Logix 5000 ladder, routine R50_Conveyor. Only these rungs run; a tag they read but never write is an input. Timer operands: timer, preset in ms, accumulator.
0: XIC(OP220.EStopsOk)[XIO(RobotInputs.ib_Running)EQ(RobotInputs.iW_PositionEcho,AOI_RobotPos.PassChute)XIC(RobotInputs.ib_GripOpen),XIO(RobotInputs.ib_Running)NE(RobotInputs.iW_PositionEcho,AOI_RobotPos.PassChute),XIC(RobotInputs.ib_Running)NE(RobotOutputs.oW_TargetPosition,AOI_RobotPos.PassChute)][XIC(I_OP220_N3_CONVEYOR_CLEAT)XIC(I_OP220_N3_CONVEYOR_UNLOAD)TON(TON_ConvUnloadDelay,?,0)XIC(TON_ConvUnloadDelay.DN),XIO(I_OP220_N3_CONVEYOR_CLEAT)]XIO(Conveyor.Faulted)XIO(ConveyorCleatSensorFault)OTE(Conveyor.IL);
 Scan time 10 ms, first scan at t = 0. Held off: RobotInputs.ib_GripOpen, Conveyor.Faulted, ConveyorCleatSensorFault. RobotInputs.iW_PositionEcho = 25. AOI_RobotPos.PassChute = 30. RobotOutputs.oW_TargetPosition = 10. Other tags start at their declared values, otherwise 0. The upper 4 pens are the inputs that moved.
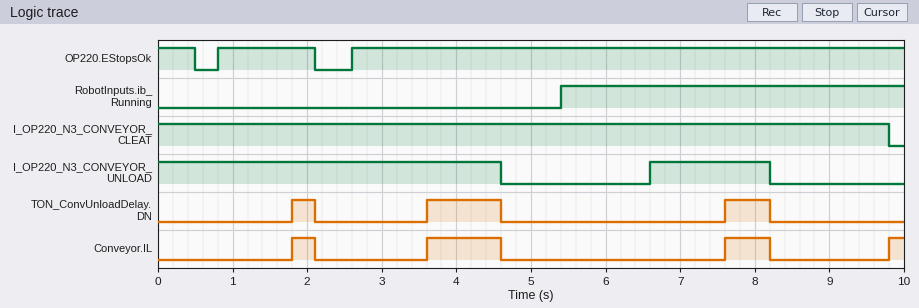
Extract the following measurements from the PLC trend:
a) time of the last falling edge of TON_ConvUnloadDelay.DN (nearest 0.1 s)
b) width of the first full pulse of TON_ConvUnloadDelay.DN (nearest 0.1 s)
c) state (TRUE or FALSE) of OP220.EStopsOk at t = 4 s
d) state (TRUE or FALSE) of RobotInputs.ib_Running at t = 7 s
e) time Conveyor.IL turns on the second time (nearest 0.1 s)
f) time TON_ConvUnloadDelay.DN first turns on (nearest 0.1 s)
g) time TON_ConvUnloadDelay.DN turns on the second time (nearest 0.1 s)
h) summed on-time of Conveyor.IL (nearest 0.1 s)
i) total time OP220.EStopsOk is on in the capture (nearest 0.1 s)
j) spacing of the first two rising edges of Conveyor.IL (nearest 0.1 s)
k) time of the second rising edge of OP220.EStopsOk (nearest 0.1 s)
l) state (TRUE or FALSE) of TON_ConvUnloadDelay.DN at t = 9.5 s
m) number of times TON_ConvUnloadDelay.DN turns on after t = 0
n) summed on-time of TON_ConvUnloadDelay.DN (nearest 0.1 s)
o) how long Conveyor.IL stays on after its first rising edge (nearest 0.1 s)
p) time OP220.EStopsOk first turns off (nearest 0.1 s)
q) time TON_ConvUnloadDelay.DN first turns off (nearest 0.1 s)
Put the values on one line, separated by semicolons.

8.2 s; 0.3 s; TRUE; TRUE; 3.6 s; 1.8 s; 3.6 s; 2.1 s; 9.2 s; 1.8 s; 2.6 s; FALSE; 3; 1.9 s; 0.3 s; 0.5 s; 2.1 s
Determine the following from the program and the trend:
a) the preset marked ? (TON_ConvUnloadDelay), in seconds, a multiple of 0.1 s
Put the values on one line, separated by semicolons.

1.0 s
